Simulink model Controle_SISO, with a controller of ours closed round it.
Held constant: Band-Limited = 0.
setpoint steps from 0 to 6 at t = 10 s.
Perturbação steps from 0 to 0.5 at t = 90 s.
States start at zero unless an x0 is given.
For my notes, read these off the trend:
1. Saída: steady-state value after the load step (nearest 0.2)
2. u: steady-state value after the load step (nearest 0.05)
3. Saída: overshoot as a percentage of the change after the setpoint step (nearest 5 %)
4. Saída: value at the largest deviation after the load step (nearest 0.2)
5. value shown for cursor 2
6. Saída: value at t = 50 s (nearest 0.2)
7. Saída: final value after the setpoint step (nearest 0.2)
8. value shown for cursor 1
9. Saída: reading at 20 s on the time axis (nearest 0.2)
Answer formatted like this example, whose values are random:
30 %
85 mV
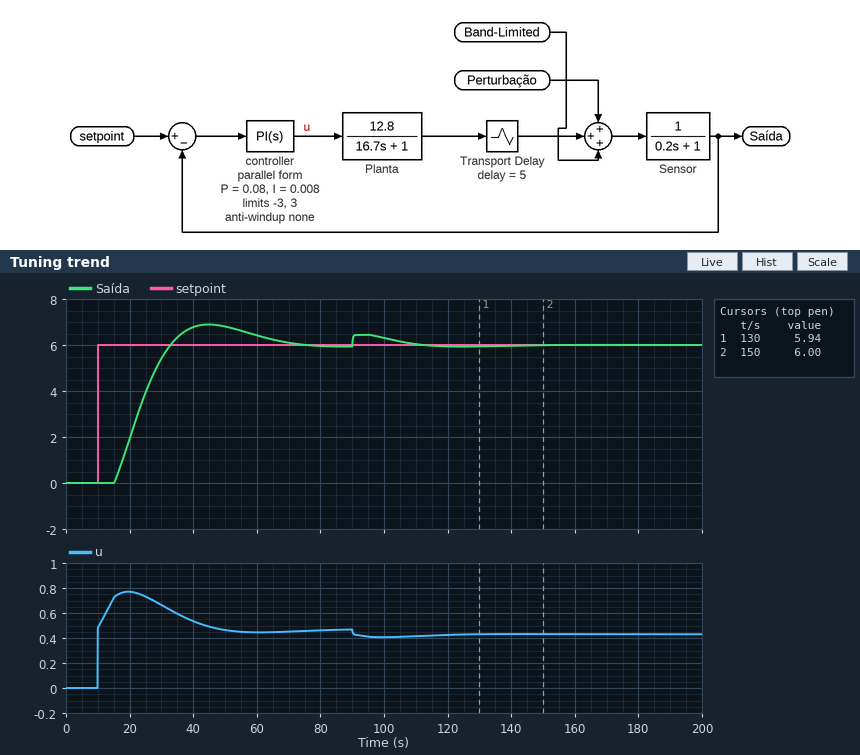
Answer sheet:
6.0
0.45
15 %
6.4
6.00
6.8
6.0
5.94
2.0
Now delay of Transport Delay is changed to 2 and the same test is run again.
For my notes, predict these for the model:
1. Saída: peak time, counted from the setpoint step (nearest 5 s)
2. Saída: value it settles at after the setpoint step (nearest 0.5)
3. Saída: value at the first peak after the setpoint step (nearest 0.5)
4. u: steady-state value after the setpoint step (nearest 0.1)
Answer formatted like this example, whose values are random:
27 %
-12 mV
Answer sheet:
40 s
6.0
6.5
0.5
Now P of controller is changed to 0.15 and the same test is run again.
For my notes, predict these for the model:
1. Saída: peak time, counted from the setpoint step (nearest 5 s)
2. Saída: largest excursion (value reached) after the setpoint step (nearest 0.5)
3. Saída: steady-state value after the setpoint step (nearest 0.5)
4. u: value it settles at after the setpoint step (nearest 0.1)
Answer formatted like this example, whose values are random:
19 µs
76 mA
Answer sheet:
20 s
6.5
6.0
0.5
